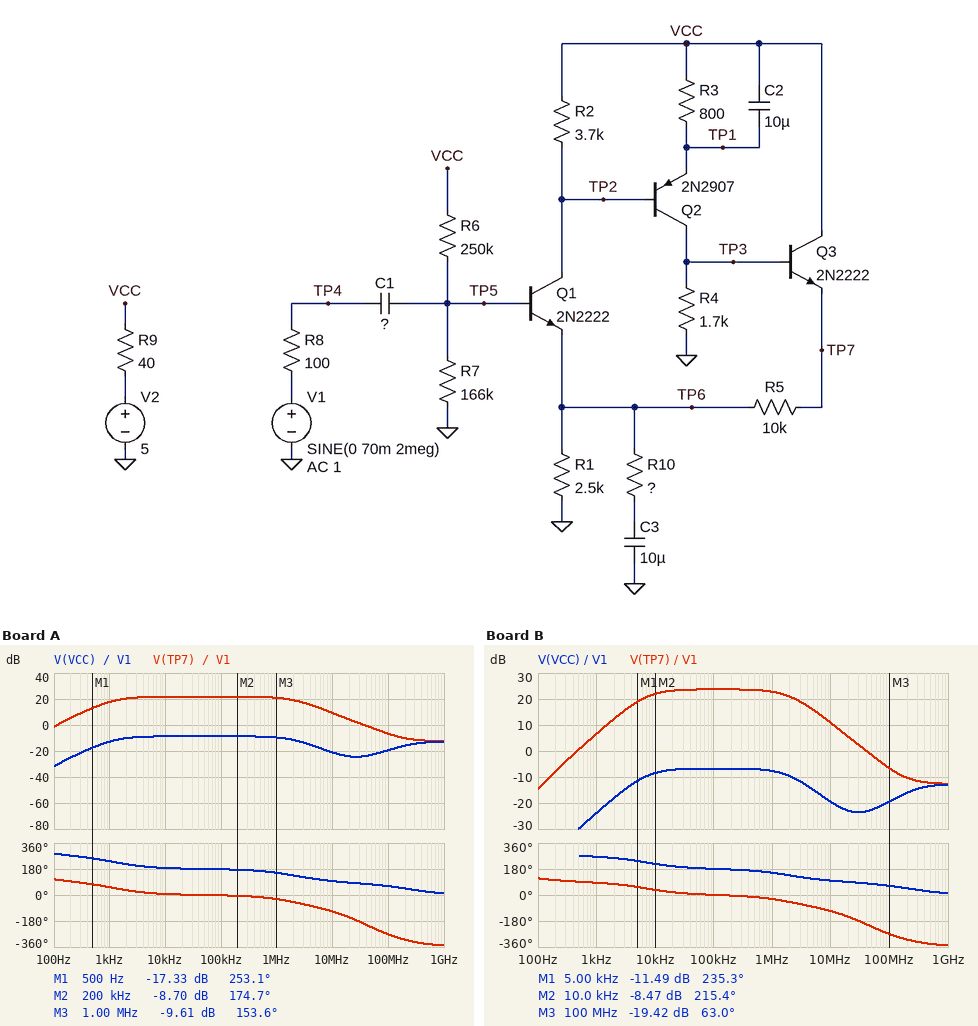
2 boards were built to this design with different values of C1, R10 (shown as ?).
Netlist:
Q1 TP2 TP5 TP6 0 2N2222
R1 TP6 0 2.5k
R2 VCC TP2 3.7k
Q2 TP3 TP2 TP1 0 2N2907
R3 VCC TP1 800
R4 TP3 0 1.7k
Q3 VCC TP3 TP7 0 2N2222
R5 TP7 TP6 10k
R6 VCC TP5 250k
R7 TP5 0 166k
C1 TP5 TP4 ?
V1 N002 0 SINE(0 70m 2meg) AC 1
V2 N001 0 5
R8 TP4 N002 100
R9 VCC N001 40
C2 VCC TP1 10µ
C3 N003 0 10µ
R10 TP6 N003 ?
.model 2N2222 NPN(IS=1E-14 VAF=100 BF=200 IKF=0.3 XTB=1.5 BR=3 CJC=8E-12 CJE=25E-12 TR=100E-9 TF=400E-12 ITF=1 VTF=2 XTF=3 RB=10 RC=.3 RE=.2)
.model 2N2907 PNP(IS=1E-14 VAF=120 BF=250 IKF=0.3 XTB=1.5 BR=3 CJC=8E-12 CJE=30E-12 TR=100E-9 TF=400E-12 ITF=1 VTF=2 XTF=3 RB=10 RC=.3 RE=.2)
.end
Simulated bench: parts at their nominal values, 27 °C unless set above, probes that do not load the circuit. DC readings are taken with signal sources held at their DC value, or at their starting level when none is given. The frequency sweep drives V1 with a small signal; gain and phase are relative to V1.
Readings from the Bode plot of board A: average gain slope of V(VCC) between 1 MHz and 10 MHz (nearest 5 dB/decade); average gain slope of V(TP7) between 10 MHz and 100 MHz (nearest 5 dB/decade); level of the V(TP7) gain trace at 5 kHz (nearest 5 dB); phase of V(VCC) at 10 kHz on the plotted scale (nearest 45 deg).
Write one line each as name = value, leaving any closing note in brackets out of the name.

average gain slope of V(VCC) between 1 MHz and 10 MHz = -10 dB/decade
average gain slope of V(TP7) between 10 MHz and 100 MHz = -15 dB/decade
level of the V(TP7) gain trace at 5 kHz = 20 dB
phase of V(VCC) at 10 kHz on the plotted scale = 180 deg
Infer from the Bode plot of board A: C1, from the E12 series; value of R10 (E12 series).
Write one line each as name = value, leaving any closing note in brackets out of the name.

C1, from the E12 series = 1.5 nF
value of R10 = 1.2 kΩ
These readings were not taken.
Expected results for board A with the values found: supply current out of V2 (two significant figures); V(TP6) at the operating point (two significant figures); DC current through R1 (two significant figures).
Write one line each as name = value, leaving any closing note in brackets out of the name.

supply current out of V2 = 1.6 mA
V(TP6) at the operating point = 1.1 V
DC current through R1 = 450 µA
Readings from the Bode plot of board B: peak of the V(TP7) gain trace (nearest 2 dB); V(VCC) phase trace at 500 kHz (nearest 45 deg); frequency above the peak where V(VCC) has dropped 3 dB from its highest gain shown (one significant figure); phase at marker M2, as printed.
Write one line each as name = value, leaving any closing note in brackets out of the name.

peak of the V(TP7) gain trace = 24 dB
V(VCC) phase trace at 500 kHz = 180 deg
frequency above the peak where V(VCC) has dropped 3 dB from its highest gain shown = 2 MHz
phase at marker M2, as printed = 215.4 deg
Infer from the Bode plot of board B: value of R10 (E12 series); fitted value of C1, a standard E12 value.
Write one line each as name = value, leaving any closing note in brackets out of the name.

value of R10 = 820 Ω
fitted value of C1, a standard E12 value = 270 pF
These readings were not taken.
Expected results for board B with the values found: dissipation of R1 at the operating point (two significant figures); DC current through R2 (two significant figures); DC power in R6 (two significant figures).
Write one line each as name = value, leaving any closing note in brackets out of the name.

dissipation of R1 at the operating point = 510 µW
DC current through R2 = 420 µA
DC power in R6 = 40 µW
